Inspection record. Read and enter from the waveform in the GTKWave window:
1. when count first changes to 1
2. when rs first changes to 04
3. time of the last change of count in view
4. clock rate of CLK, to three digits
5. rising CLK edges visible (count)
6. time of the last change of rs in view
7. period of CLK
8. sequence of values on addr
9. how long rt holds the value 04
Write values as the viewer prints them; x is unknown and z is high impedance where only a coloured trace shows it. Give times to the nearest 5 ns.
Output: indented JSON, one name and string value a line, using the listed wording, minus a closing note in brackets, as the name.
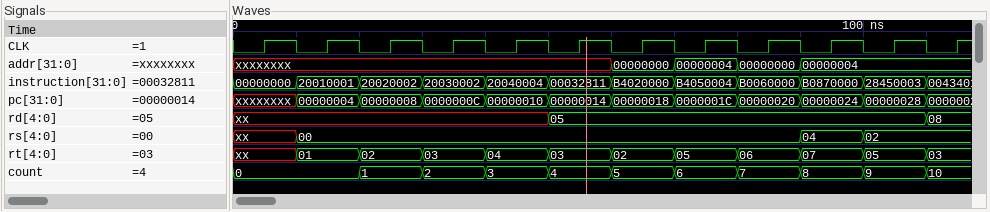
{
  "when count first changes to 1": "20 ns",
  "when rs first changes to 04": "90 ns",
  "time of the last change of count in view": "110 ns",
  "clock rate of CLK, to three digits": "100 MHz",
  "rising CLK edges visible": "12",
  "time of the last change of rs in view": "100 ns",
  "period of CLK": "10 ns",
  "sequence of values on addr": "xxxxxxxx, 00000000, 00000004, 00000000, 00000004",
  "how long rt holds the value 04": "10 ns"
}
